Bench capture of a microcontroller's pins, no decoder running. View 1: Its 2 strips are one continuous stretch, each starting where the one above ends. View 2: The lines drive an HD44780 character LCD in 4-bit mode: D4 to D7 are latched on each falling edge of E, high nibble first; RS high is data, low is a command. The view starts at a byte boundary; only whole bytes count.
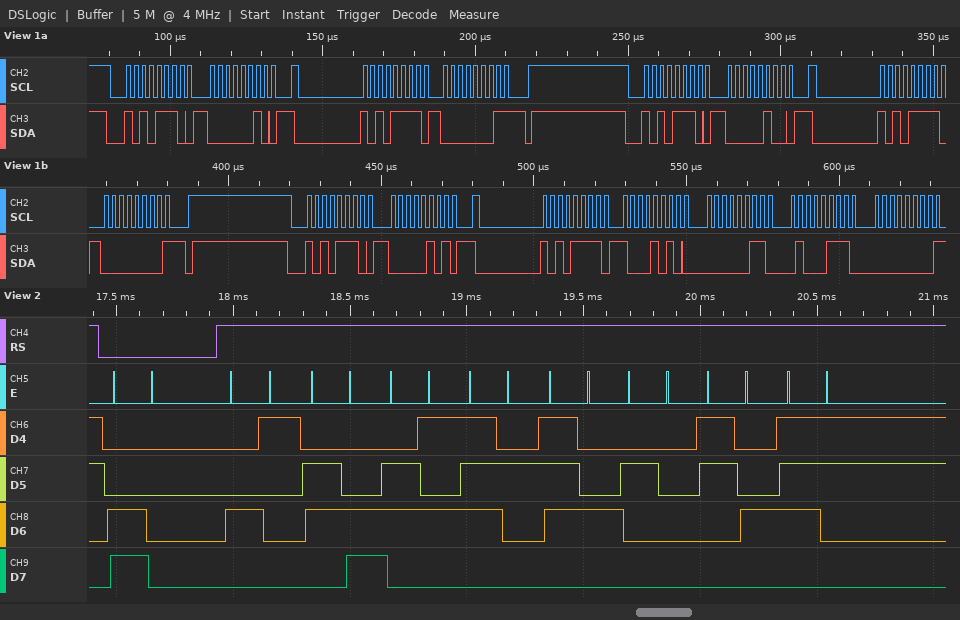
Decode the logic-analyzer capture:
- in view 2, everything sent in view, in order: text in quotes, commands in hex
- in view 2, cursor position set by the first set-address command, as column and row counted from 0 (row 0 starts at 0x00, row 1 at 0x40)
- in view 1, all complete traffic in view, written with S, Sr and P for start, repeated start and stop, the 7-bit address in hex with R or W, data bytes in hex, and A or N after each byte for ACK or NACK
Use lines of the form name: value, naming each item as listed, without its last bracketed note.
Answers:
in view 2, everything sent in view, in order: text in quotes, commands in hex: 0xC0 "Alert 4s"
in view 2, cursor position set by the first set-address command, as column and row counted from 0: column 0, row 1
in view 1, all complete traffic in view, written with S, Sr and P for start, repeated start and stop, the 7-bit address in hex with R or W, data bytes in hex, and A or N after each byte for ACK or NACK: S 57W A 02 A Sr 57R A 01 N P S 57W A 04 A Sr 57R A 00 N P S 57W A 05 A Sr 57R A 8A A 03 A 47 A 00 N
